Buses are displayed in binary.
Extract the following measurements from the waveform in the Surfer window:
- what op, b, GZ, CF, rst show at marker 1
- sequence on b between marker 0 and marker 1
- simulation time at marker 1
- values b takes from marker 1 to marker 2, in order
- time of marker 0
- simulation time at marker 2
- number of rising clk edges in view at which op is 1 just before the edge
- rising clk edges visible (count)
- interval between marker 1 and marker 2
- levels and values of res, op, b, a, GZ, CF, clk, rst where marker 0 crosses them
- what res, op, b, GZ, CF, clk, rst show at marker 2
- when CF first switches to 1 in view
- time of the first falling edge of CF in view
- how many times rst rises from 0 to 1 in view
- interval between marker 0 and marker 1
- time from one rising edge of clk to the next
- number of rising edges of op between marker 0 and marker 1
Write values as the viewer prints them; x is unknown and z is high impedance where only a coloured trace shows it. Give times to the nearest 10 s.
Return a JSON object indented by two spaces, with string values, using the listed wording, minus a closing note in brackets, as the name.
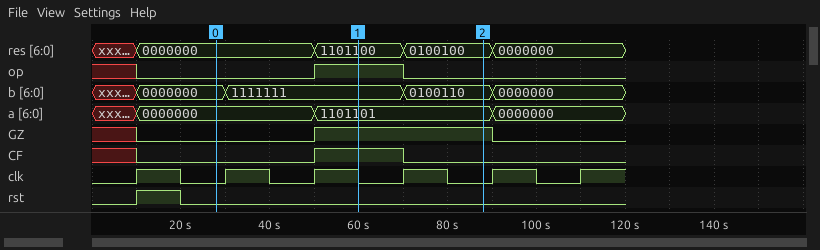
{
  "what op, b, GZ, CF, rst show at marker 1": "op=1, b=1111111, GZ=1, CF=1, rst=0",
  "sequence on b between marker 0 and marker 1": "0000000, 1111111",
  "simulation time at marker 1": "60 s",
  "values b takes from marker 1 to marker 2, in order": "1111111, 0100110",
  "time of marker 0": "30 s",
  "simulation time at marker 2": "90 s",
  "number of rising clk edges in view at which op is 1 just before the edge": "1",
  "rising clk edges visible": "6",
  "interval between marker 1 and marker 2": "30 s",
  "levels and values of res, op, b, a, GZ, CF, clk, rst where marker 0 crosses them": "res=0000000, op=0, b=0000000, a=0000000, GZ=0, CF=0, clk=0, rst=0",
  "what res, op, b, GZ, CF, clk, rst show at marker 2": "res=0100100, op=0, b=0100110, GZ=1, CF=0, clk=0, rst=0",
  "when CF first switches to 1 in view": "50 s",
  "time of the first falling edge of CF in view": "70 s",
  "how many times rst rises from 0 to 1 in view": "1",
  "interval between marker 0 and marker 1": "30 s",
  "time from one rising edge of clk to the next": "20 s",
  "number of rising edges of op between marker 0 and marker 1": "1"
}
